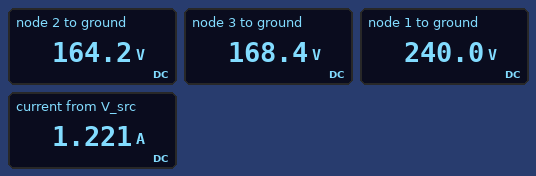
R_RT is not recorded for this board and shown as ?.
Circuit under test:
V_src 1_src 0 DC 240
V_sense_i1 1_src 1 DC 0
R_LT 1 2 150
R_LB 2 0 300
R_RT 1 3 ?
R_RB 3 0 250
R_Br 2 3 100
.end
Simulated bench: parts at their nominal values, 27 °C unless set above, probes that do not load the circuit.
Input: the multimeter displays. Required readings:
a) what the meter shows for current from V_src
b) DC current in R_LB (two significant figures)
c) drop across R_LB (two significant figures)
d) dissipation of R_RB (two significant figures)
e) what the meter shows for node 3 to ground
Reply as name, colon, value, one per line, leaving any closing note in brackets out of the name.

what the meter shows for current from V_src: 1.221 A
DC current in R_LB: 550 mA
drop across R_LB: 160 V
dissipation of R_RB: 110 W
what the meter shows for node 3 to ground: 168.4 V
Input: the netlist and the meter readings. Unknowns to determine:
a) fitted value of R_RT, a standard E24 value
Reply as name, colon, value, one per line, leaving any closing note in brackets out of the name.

fitted value of R_RT, a standard E24 value: 100 Ω
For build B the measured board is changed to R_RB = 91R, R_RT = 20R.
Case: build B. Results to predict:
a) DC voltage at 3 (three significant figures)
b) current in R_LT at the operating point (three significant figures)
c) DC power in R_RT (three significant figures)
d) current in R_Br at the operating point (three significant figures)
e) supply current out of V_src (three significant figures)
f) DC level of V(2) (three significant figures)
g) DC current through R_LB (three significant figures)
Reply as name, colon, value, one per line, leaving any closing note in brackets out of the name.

DC voltage at 3: 194 V
current in R_LT at the operating point: 420 mA
DC power in R_RT: 106 W
current in R_Br at the operating point: 170 mA
supply current out of V_src: 2.72 A
DC level of V(2): 177 V
DC current through R_LB: 590 mA
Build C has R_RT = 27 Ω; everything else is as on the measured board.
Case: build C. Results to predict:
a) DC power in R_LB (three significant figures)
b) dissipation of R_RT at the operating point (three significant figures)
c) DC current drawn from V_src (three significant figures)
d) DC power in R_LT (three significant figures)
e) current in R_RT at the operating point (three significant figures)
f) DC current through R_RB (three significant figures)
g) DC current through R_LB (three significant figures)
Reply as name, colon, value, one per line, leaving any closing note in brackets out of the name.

DC power in R_LB: 114 W
dissipation of R_RT at the operating point: 32.3 W
DC current drawn from V_src: 1.46 A
DC power in R_LT: 20.0 W
current in R_RT at the operating point: 1.09 A
DC current through R_RB: 842 mA
DC current through R_LB: 617 mA
